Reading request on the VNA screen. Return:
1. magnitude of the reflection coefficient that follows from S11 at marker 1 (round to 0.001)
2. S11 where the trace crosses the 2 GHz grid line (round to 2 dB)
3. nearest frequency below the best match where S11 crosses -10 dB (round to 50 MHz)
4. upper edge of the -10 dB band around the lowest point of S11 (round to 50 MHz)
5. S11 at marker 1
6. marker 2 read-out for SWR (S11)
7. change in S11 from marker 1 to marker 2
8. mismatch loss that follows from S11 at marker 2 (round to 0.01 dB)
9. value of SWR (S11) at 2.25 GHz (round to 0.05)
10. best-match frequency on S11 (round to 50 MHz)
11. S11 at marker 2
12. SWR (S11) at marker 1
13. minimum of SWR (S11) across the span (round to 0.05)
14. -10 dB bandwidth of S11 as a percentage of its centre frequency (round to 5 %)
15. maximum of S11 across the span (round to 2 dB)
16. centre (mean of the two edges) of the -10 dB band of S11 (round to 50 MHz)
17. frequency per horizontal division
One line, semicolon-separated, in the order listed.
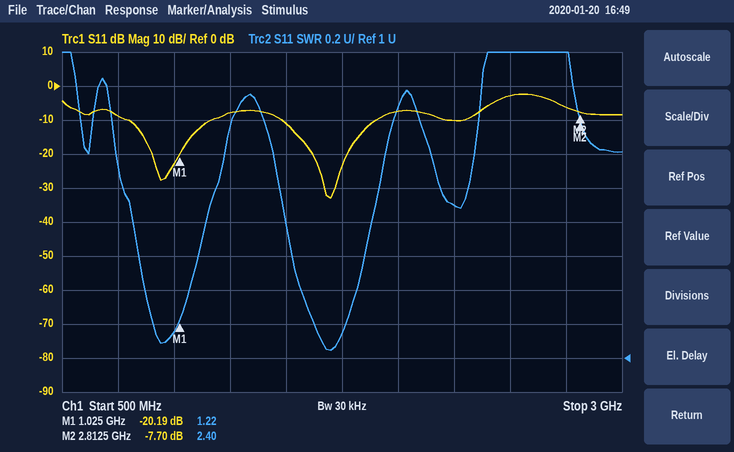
0.098; -8 dB; 1.50 GHz; 1.90 GHz; -20.19 dB; 2.40; 12.49 dB; 0.81 dB; 1.90; 1.70 GHz; -7.70 dB; 1.22; 1.05; 25 %; -2 dB; 1.70 GHz; 250 MHz
